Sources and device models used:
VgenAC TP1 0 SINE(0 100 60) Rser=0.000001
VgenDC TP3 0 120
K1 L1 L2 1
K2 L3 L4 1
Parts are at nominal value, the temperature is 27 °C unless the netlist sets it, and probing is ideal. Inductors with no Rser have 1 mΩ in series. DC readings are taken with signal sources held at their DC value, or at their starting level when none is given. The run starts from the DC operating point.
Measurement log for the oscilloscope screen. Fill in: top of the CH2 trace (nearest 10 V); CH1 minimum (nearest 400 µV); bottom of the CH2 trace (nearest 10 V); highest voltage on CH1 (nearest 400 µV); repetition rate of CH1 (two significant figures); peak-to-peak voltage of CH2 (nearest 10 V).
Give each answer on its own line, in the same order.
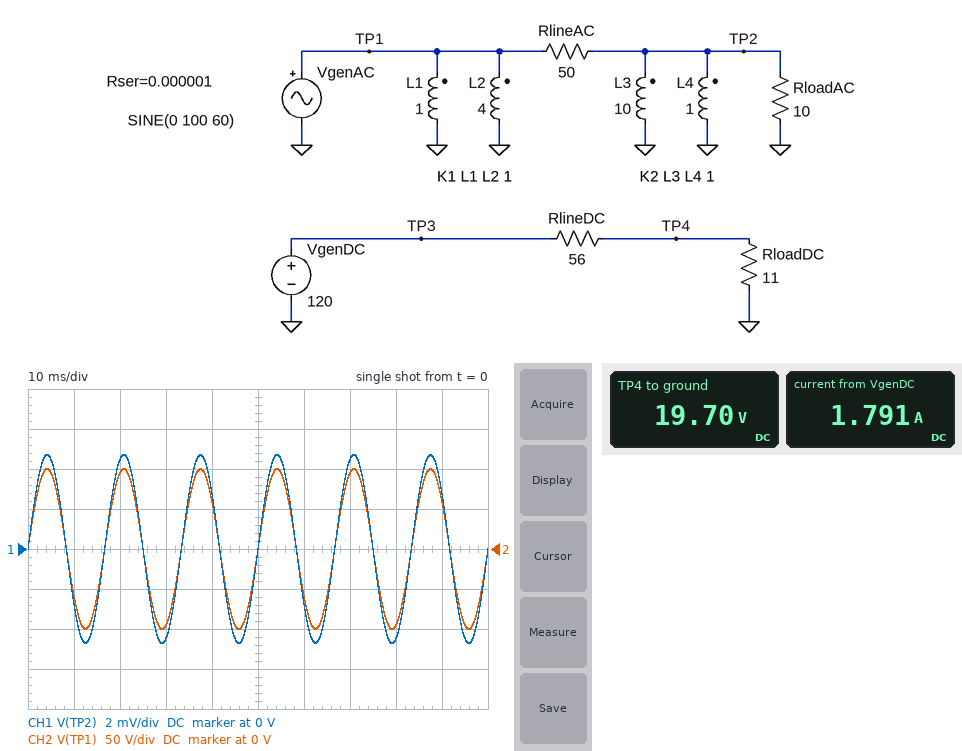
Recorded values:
100 V
-4.8 mV
-100 V
4.8 mV
60 Hz
200 V
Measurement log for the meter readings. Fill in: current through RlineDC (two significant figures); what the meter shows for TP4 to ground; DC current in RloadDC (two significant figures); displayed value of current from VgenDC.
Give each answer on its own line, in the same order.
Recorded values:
1.8 A
19.70 V
1.8 A
1.791 A
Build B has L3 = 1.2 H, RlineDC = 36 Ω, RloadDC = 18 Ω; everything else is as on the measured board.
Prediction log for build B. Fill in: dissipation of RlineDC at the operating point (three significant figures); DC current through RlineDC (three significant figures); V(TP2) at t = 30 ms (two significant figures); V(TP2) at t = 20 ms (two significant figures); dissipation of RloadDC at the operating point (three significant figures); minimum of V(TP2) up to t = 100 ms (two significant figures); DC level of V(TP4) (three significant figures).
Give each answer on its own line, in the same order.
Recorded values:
178 W
2.22 A
-450 mV
450 mV
88.9 W
-470 mV
40.0 V
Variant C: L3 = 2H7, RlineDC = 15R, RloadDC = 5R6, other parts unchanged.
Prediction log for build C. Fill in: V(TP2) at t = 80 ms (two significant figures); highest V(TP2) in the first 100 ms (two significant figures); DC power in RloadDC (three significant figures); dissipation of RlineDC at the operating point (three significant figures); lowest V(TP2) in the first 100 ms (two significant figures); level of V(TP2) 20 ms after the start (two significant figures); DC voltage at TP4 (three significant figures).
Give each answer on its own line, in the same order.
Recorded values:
-17 mV
18 mV
190 W
509 W
-18 mV
17 mV
32.6 V
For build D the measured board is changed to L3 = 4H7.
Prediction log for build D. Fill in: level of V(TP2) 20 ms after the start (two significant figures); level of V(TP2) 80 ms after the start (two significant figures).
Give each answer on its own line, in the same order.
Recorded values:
7.9 mV
-7.9 mV
